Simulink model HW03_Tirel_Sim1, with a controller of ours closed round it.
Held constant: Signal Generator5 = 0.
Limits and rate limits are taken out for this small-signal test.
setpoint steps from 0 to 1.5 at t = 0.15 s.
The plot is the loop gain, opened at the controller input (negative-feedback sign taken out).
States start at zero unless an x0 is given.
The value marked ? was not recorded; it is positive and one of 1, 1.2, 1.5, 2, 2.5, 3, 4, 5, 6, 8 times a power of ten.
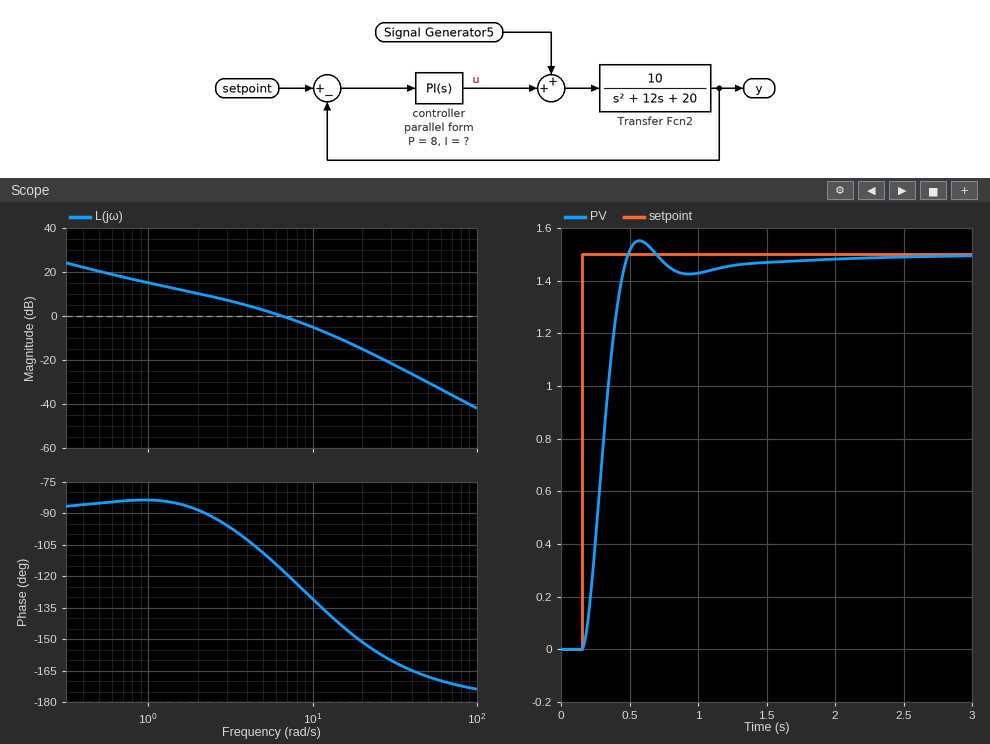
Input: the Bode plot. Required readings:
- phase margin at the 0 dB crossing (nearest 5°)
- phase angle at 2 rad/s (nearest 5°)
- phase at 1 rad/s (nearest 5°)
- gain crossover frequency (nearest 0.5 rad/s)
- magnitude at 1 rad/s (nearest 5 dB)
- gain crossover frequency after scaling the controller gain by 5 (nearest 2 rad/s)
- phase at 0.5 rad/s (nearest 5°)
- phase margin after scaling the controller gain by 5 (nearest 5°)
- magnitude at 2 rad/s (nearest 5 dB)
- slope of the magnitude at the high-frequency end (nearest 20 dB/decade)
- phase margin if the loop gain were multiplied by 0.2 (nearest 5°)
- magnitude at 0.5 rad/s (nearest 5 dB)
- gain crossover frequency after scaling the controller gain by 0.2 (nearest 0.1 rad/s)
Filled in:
65°
-90°
-85°
6.5 rad/s
15 dB
18 rad/s
-85°
30°
10 dB
-40 dB/decade
95°
20 dB
1.2 rad/s
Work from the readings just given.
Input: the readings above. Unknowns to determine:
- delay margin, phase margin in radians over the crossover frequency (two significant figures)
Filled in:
0.17 s
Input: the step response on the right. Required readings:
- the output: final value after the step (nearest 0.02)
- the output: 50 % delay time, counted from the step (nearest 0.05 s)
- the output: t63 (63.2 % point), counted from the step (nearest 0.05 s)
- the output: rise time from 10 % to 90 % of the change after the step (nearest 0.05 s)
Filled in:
1.50
0.15 s
0.20 s
0.20 s
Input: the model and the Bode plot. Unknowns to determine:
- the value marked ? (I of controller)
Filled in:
10
